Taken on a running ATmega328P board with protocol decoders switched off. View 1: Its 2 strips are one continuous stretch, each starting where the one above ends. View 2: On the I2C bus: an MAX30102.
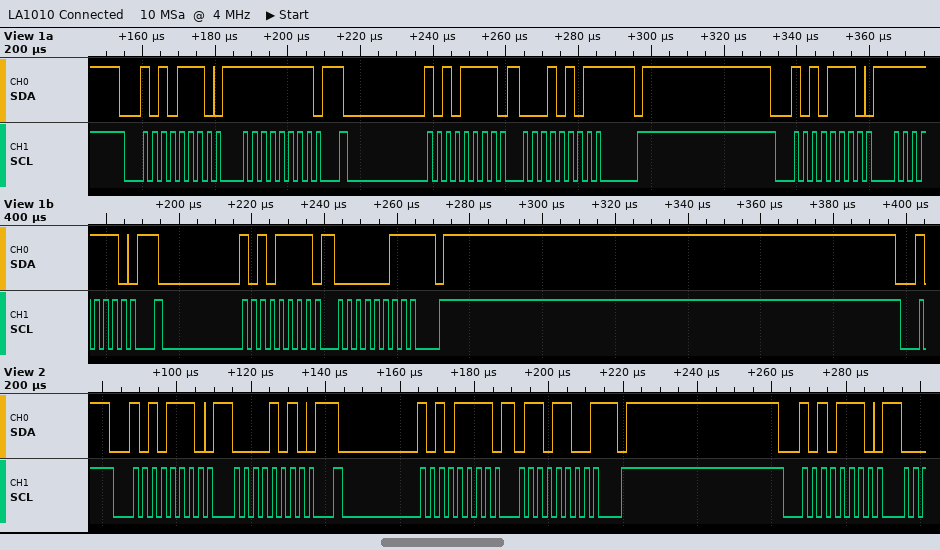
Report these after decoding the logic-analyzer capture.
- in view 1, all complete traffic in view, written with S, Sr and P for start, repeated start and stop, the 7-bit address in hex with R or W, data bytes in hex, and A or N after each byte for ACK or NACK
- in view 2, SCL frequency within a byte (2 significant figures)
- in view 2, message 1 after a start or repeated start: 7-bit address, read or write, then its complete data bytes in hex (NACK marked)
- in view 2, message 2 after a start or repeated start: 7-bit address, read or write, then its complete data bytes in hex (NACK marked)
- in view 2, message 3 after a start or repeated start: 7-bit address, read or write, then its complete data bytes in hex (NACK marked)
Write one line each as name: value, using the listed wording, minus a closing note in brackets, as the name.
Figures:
in view 1, all complete traffic in view, written with S, Sr and P for start, repeated start and stop, the 7-bit address in hex with R or W, data bytes in hex, and A or N after each byte for ACK or NACK: S 57W A FF A Sr 57R A 15 N P S 57W A FE A Sr 57R A 03 N P
in view 2, SCL frequency within a byte: 400 kHz
in view 2, message 1 after a start or repeated start: 7-bit address, read or write, then its complete data bytes in hex: 0x57 write: 0A
in view 2, message 2 after a start or repeated start: 7-bit address, read or write, then its complete data bytes in hex: 0x57 read: 6C NACK
in view 2, message 3 after a start or repeated start: 7-bit address, read or write, then its complete data bytes in hex: 0x57 write
